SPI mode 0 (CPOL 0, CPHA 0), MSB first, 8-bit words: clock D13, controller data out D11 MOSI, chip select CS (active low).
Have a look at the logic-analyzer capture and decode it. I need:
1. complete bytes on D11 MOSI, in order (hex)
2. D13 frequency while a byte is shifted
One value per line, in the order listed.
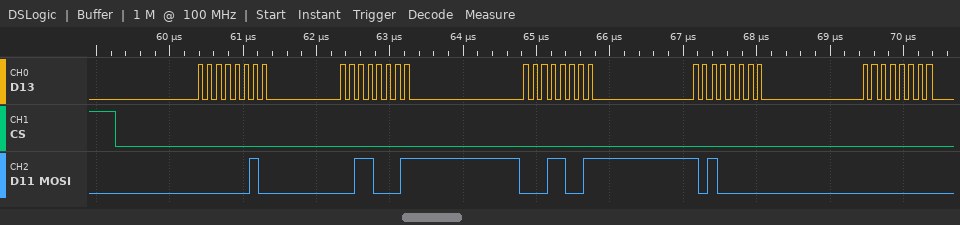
02 31 19 A0 00
8 MHz
